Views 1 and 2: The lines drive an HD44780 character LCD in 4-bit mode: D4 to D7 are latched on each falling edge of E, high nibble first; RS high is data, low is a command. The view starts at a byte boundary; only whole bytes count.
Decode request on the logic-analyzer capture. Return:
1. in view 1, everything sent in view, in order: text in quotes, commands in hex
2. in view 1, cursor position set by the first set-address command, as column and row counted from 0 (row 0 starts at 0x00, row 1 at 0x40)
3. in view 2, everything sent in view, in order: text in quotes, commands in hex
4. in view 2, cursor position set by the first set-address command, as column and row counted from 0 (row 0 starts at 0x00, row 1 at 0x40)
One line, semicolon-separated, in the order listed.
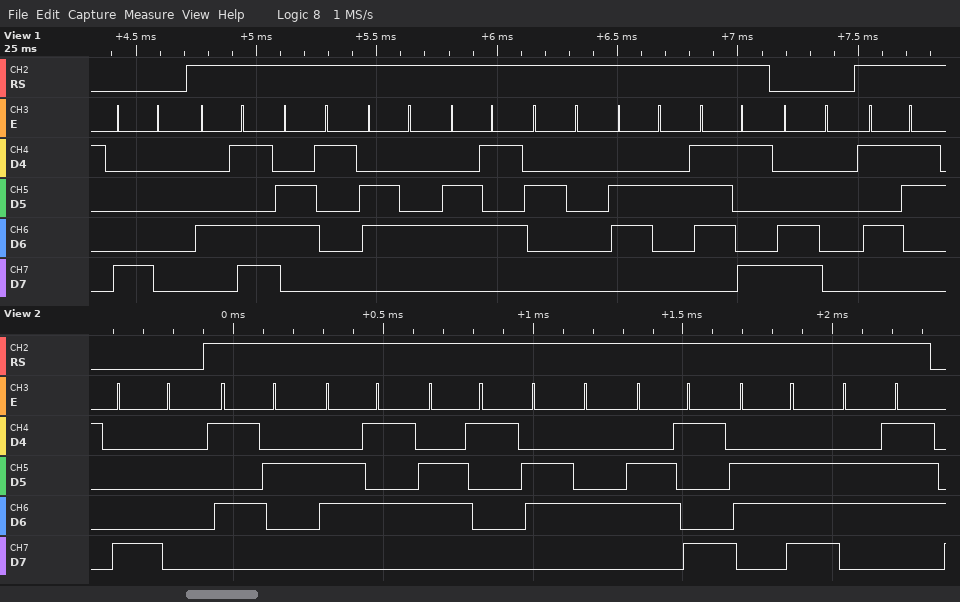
0x80 "Made by" 0xC0 "S"; column 0, row 0; 0x80 "Reading"; column 0, row 0
